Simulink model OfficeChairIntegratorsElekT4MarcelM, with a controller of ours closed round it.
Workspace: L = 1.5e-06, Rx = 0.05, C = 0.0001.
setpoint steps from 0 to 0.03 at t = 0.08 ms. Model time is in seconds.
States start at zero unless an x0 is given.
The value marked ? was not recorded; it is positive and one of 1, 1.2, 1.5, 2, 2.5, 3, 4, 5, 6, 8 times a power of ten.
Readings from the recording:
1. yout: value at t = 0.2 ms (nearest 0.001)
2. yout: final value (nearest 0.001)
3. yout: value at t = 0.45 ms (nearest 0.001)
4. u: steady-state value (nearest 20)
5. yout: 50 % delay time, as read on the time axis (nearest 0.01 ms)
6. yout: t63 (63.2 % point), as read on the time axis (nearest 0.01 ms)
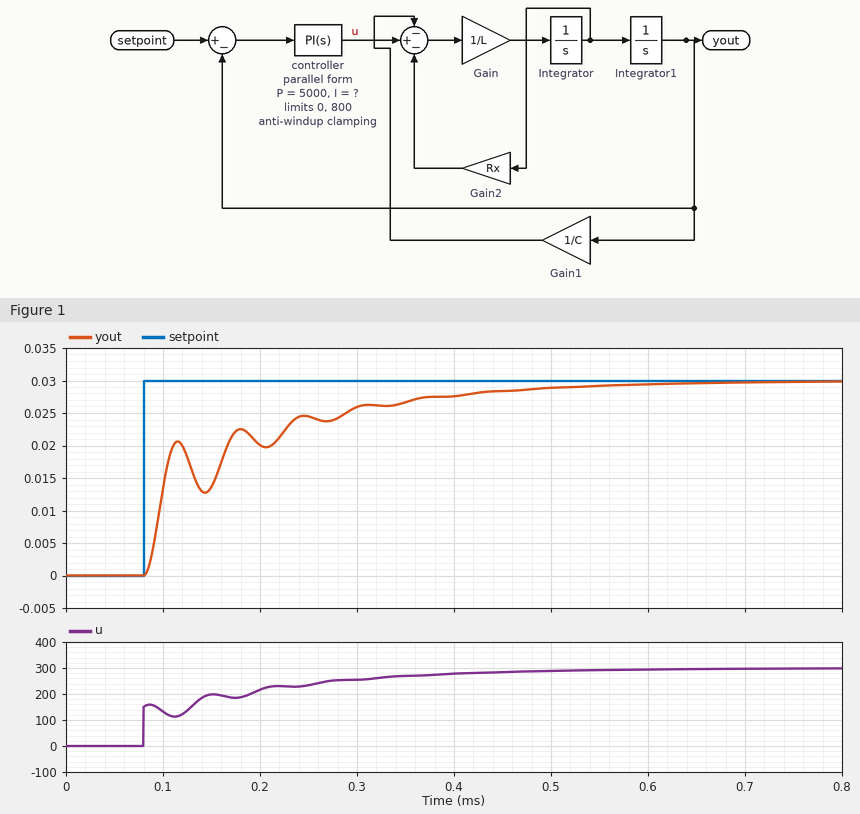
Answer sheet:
0.020
0.030
0.028
300
0.10 ms
0.11 ms
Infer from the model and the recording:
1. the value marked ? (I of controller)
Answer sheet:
1e+08
